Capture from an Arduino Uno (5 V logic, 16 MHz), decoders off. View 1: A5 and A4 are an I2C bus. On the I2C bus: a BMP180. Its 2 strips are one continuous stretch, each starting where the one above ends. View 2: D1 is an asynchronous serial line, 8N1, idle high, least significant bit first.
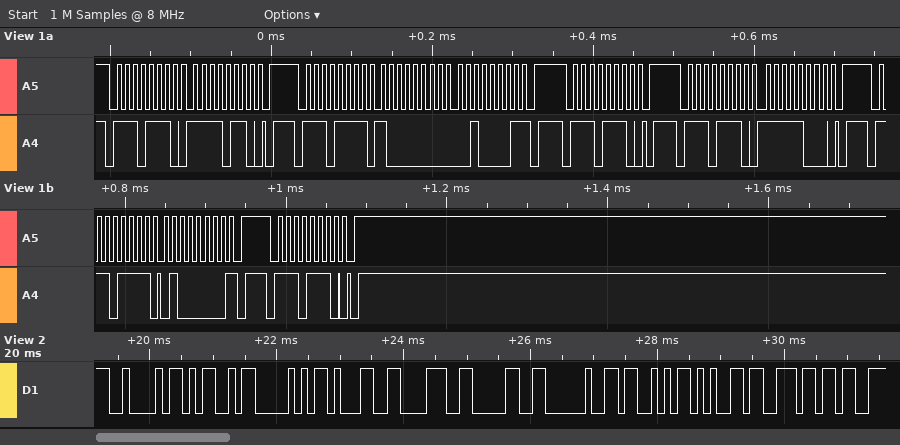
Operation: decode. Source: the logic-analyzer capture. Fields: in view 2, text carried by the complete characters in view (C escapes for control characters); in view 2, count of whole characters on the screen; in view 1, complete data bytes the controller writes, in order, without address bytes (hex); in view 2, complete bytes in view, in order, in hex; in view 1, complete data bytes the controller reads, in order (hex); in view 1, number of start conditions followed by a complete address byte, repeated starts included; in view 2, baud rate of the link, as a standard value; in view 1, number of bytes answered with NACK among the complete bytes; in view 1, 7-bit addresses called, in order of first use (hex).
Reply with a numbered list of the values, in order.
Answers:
1. "BMP180 Sen"
2. 10
3. F6 F8
4. 42 4D 50 31 38 30 20 53 65 6E
5. 80 21 40
6. 6
7. 9600 baud
8. 2
9. 0x77
